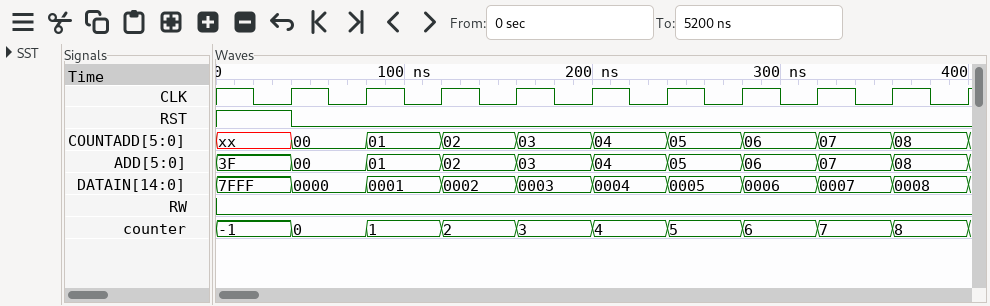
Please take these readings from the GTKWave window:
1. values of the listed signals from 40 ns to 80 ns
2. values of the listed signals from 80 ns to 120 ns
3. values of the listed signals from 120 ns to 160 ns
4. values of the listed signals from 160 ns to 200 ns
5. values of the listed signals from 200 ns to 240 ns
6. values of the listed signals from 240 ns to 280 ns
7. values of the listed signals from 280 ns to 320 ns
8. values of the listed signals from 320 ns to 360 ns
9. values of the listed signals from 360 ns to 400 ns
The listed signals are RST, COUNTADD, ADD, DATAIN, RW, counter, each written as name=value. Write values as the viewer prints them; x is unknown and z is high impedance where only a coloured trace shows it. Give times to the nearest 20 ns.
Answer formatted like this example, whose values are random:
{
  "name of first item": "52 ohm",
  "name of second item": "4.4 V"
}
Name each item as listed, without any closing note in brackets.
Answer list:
{
  "values of the listed signals from 40 ns to 80 ns": "RST=0, COUNTADD=00, ADD=00, DATAIN=0000, RW=0, counter=0",
  "values of the listed signals from 80 ns to 120 ns": "RST=0, COUNTADD=01, ADD=01, DATAIN=0001, RW=0, counter=1",
  "values of the listed signals from 120 ns to 160 ns": "RST=0, COUNTADD=02, ADD=02, DATAIN=0002, RW=0, counter=2",
  "values of the listed signals from 160 ns to 200 ns": "RST=0, COUNTADD=03, ADD=03, DATAIN=0003, RW=0, counter=3",
  "values of the listed signals from 200 ns to 240 ns": "RST=0, COUNTADD=04, ADD=04, DATAIN=0004, RW=0, counter=4",
  "values of the listed signals from 240 ns to 280 ns": "RST=0, COUNTADD=05, ADD=05, DATAIN=0005, RW=0, counter=5",
  "values of the listed signals from 280 ns to 320 ns": "RST=0, COUNTADD=06, ADD=06, DATAIN=0006, RW=0, counter=6",
  "values of the listed signals from 320 ns to 360 ns": "RST=0, COUNTADD=07, ADD=07, DATAIN=0007, RW=0, counter=7",
  "values of the listed signals from 360 ns to 400 ns": "RST=0, COUNTADD=08, ADD=08, DATAIN=0008, RW=0, counter=8"
}
